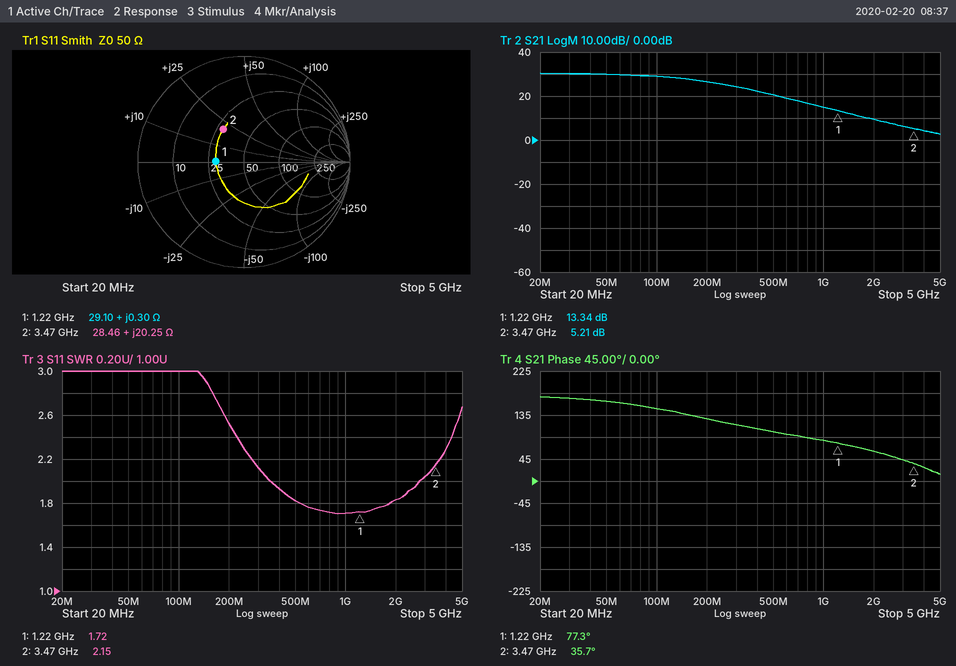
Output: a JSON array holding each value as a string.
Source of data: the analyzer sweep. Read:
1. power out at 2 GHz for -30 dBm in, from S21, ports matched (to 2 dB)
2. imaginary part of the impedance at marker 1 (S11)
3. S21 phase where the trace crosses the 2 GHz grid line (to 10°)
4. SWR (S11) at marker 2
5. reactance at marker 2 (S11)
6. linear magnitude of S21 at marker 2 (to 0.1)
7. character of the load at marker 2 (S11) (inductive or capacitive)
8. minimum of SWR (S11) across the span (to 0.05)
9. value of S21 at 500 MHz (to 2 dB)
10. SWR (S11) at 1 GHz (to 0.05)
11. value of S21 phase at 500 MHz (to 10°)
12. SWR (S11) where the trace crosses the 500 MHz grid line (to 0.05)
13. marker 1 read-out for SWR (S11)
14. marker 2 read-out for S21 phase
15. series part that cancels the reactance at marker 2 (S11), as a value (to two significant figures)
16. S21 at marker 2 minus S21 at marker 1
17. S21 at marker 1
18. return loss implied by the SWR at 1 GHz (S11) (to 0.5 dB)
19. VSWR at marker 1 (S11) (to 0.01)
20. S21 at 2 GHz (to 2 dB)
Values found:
["-20 dBm", "+0.30 Ω", "60°", "2.15", "+20.25 Ω", "1.8", "inductive", "1.70", "20 dB", "1.70", "100°", "1.80", "1.72", "35.7°", "2.3 pF", "-8.13 dB", "13.34 dB", "11.5 dB", "1.72", "10 dB"]
